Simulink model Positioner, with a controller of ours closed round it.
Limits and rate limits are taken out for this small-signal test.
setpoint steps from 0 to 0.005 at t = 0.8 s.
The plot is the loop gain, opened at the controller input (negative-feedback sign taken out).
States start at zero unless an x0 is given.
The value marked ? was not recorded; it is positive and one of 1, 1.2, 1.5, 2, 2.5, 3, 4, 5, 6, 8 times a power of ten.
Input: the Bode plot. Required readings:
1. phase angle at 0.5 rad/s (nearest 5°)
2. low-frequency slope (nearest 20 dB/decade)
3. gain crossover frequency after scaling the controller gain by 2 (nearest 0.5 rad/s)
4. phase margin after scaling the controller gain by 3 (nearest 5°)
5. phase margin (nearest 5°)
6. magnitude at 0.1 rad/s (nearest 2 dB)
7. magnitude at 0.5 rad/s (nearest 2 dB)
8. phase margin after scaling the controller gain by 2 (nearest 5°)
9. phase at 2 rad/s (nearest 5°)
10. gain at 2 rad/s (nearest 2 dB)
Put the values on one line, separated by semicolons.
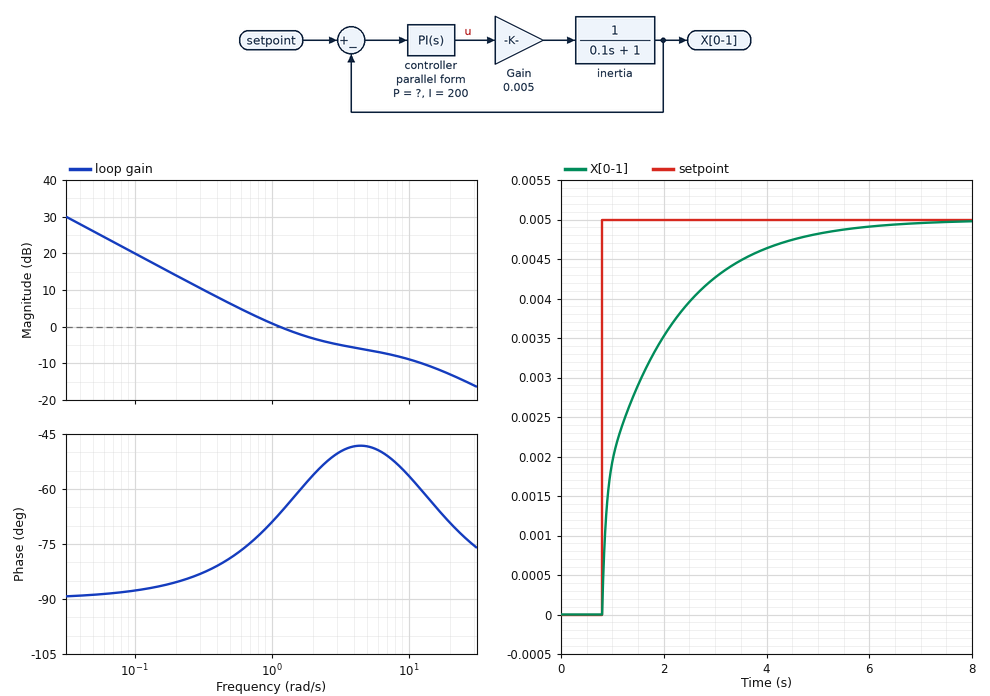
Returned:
-80°; -20 dB/decade; 4.5 rad/s; 120°; 115°; 20 dB; 6 dB; 130°; -55°; -4 dB
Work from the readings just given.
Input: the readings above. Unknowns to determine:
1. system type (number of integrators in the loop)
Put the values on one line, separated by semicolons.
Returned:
1
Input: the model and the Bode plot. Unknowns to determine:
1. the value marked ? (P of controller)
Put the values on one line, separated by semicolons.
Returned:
100
